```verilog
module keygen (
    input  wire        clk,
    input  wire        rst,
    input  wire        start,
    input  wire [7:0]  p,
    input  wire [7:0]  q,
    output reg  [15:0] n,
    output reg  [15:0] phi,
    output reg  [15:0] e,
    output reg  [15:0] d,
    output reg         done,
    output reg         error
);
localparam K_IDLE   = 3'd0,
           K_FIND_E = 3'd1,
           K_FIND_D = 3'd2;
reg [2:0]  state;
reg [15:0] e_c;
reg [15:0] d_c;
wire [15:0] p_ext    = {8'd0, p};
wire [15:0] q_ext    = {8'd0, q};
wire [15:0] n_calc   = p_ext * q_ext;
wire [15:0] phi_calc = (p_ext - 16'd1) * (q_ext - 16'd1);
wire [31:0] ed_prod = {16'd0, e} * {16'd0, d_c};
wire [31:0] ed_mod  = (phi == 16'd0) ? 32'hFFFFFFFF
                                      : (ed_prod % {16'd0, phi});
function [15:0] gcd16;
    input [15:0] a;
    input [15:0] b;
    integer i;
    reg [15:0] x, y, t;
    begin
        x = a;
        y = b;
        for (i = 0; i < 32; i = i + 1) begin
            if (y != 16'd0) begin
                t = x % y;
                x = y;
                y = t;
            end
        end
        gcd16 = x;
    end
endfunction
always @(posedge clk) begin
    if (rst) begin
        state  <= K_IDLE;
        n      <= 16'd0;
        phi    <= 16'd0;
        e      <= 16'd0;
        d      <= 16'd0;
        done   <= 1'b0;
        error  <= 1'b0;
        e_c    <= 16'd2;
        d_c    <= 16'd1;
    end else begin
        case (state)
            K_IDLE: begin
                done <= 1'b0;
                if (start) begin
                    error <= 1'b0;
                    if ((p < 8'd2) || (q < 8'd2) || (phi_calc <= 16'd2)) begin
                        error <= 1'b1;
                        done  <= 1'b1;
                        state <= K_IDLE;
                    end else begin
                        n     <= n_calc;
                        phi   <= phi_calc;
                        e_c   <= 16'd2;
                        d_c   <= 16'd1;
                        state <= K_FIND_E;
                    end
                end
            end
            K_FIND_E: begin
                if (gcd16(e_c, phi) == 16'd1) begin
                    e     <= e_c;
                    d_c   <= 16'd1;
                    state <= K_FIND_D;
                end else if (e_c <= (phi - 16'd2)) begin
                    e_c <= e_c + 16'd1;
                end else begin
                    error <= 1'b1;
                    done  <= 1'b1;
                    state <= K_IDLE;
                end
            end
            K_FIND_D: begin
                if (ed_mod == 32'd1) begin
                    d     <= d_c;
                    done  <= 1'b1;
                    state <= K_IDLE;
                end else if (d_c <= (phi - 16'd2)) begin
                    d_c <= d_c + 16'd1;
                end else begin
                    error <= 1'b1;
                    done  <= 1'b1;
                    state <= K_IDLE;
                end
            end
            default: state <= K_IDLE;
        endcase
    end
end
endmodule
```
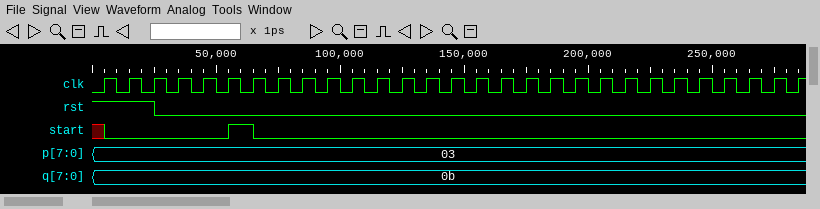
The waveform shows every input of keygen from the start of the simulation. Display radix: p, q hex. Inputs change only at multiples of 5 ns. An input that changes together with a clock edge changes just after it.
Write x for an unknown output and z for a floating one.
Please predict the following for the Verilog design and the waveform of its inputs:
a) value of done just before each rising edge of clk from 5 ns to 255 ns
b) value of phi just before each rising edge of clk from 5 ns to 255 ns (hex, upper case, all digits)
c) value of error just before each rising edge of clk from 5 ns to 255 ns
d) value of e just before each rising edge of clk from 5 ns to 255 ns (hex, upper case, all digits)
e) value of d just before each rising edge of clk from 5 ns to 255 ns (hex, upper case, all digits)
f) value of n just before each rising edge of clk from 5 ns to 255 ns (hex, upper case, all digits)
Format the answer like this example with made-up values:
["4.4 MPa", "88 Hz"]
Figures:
["x 0 0 0 0 0 0 0 0 0 0 0 0 0 0 0 1 0 0 0 0 0 0 0 0 0", "x, 0000, 0000, 0000, 0000, 0000, 0000, 0014, 0014, 0014, 0014, 0014, 0014, 0014, 0014, 0014, 0014, 0014, 0014, 0014, 0014, 0014, 0014, 0014, 0014, 0014", "x 0 0 0 0 0 0 0 0 0 0 0 0 0 0 0 0 0 0 0 0 0 0 0 0 0", "x, 0000, 0000, 0000, 0000, 0000, 0000, 0000, 0000, 0003, 0003, 0003, 0003, 0003, 0003, 0003, 0003, 0003, 0003, 0003, 0003, 0003, 0003, 0003, 0003, 0003", "x, 0000, 0000, 0000, 0000, 0000, 0000, 0000, 0000, 0000, 0000, 0000, 0000, 0000, 0000, 0000, 0007, 0007, 0007, 0007, 0007, 0007, 0007, 0007, 0007, 0007", "x, 0000, 0000, 0000, 0000, 0000, 0000, 0021, 0021, 0021, 0021, 0021, 0021, 0021, 0021, 0021, 0021, 0021, 0021, 0021, 0021, 0021, 0021, 0021, 0021, 0021"]
